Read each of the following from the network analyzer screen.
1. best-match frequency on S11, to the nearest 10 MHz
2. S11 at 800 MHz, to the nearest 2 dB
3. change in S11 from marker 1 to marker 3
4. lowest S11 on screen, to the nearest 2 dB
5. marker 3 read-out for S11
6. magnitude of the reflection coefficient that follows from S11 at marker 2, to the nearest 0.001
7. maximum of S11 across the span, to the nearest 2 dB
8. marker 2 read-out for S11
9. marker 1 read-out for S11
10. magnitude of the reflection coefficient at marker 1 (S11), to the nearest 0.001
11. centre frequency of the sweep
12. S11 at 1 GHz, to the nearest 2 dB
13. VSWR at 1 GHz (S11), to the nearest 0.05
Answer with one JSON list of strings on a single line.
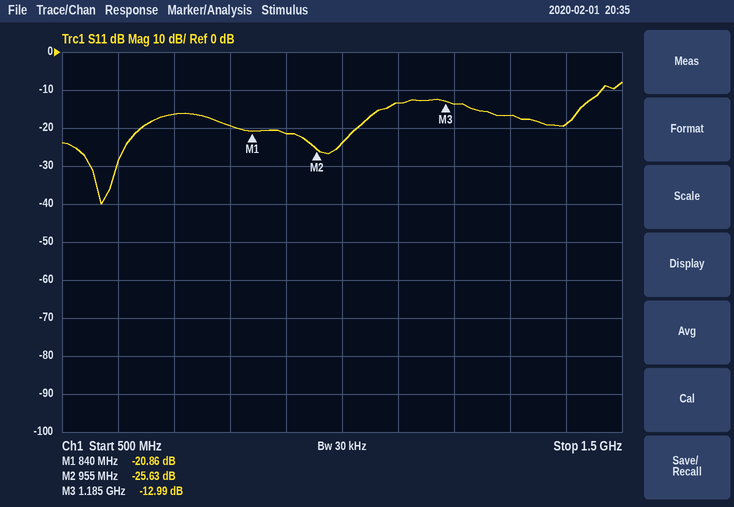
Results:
["570 MHz", "-20 dB", "7.87 dB", "-40 dB", "-12.99 dB", "0.052", "-8 dB", "-25.63 dB", "-20.86 dB", "0.091", "1 GHz", "-24 dB", "1.15"]
